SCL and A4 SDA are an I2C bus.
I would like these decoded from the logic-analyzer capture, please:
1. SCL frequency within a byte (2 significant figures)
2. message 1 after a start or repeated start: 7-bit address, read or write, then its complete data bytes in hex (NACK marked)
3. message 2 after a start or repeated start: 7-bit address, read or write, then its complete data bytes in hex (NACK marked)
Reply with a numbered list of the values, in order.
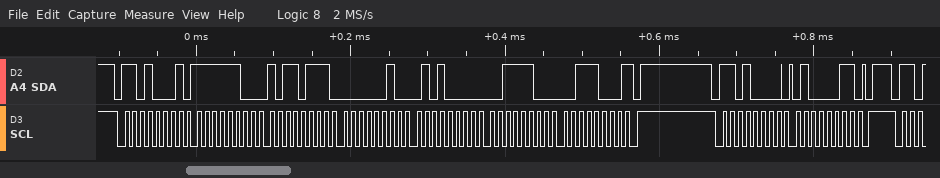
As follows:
1. 100 kHz
2. 0x68 read: FC B7 02 50 3C 38 NACK
3. 0x68 write: 43
